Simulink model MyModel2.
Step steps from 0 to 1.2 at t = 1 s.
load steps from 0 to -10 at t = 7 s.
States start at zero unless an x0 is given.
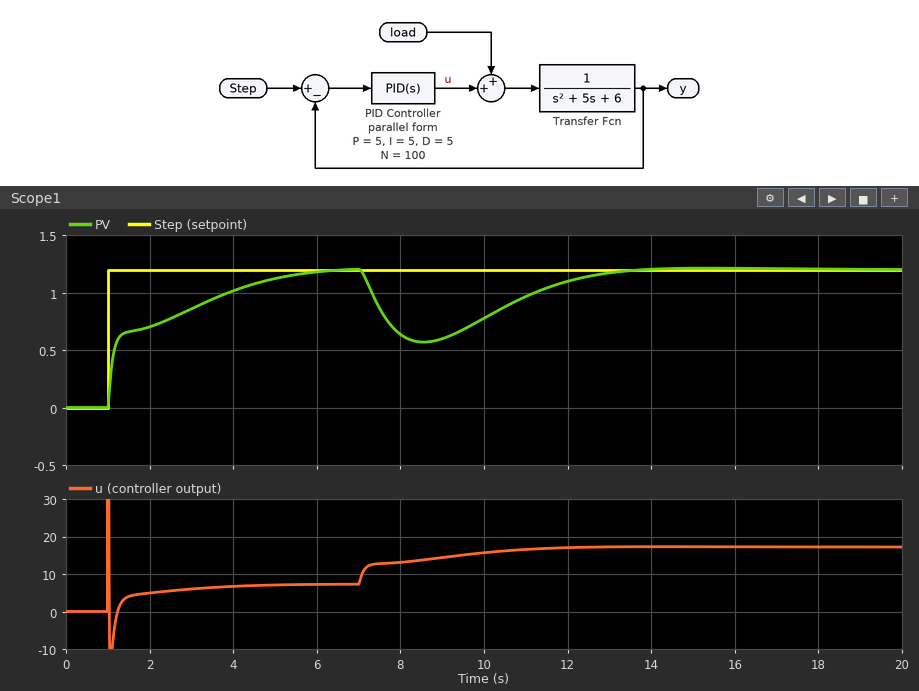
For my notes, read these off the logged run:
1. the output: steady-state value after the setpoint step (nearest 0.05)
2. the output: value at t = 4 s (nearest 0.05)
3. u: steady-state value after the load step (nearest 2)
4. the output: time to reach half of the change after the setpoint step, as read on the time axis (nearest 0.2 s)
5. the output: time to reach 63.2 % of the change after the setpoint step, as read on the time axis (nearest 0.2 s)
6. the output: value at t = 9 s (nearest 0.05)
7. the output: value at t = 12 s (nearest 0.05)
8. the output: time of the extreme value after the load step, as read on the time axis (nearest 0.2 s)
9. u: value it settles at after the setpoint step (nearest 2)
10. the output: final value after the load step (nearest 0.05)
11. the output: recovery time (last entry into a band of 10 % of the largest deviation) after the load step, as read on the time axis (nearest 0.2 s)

1.20
1.00
18
1.2 s
2.4 s
0.60
1.10
8.6 s
8
1.20
12.4 s
